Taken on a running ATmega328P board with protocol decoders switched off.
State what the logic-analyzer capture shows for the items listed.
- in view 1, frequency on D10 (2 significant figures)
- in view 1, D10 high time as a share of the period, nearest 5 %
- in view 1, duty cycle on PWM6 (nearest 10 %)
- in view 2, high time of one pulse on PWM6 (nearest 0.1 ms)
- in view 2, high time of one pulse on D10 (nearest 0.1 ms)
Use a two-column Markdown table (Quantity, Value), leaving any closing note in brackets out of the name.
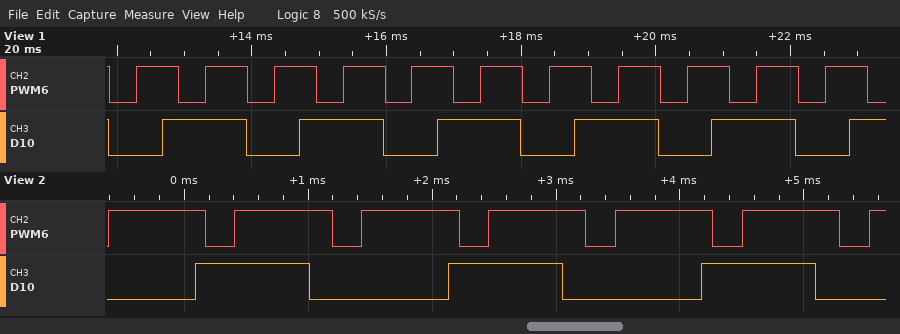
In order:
| Quantity | Value |
|---|---|
| in view 1, frequency on D10 | 490 Hz |
| in view 1, D10 high time as a share of the period, nearest 5 % | 60 % |
| in view 1, duty cycle on PWM6 | 60 % |
| in view 2, high time of one pulse on PWM6 | 0.8 ms |
| in view 2, high time of one pulse on D10 | 0.9 ms |
